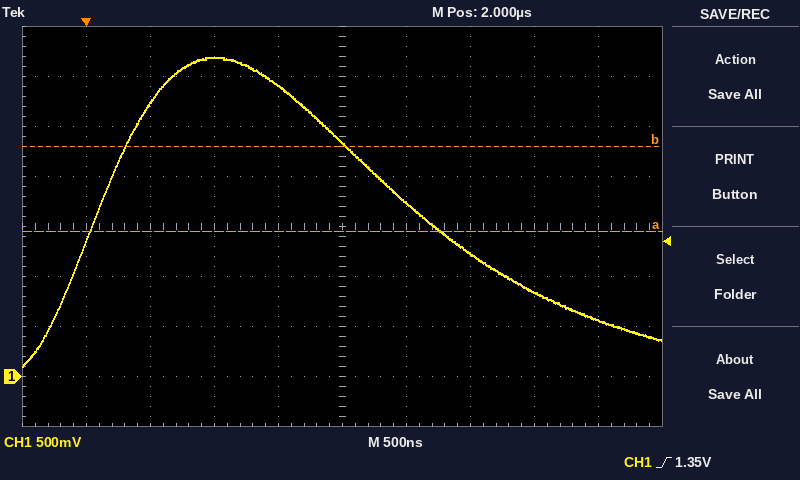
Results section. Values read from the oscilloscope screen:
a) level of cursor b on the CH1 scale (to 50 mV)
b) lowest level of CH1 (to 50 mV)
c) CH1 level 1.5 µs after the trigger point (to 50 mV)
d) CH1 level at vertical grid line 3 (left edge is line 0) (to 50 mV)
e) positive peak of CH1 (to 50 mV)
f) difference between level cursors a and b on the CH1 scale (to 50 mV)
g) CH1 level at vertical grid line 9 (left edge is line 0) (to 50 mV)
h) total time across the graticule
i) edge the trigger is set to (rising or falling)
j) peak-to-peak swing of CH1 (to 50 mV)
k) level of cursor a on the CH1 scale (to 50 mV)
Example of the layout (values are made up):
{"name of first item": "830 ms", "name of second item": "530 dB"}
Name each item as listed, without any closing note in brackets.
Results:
{"level of cursor b on the CH1 scale": "2.30 V", "lowest level of CH1": "100 mV", "CH1 level 1.5 µs after the trigger point": "2.90 V", "CH1 level at vertical grid line 3 (left edge is line 0)": "3.20 V", "positive peak of CH1": "3.20 V", "difference between level cursors a and b on the CH1 scale": "850 mV", "CH1 level at vertical grid line 9 (left edge is line 0)": "550 mV", "total time across the graticule": "5 µs", "edge the trigger is set to": "rising", "peak-to-peak swing of CH1": "3.10 V", "level of cursor a on the CH1 scale": "1.45 V"}
